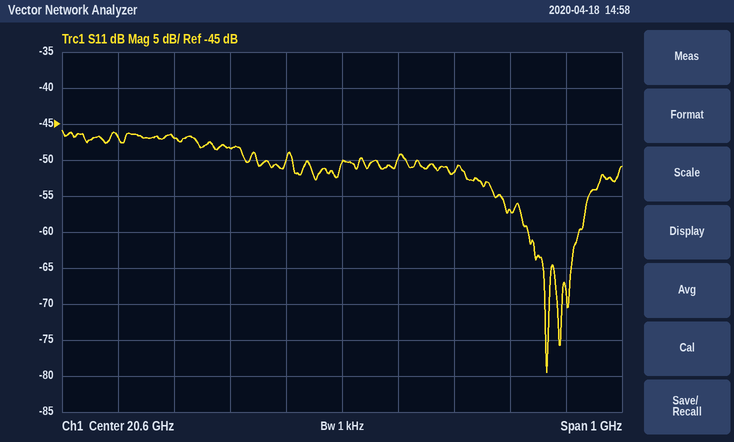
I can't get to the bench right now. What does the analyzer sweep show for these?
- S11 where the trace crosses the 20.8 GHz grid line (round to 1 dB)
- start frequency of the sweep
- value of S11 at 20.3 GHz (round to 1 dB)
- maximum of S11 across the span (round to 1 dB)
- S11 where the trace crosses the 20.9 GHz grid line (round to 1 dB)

-52 dB
20.1 GHz
-47 dB
-46 dB
-57 dB
